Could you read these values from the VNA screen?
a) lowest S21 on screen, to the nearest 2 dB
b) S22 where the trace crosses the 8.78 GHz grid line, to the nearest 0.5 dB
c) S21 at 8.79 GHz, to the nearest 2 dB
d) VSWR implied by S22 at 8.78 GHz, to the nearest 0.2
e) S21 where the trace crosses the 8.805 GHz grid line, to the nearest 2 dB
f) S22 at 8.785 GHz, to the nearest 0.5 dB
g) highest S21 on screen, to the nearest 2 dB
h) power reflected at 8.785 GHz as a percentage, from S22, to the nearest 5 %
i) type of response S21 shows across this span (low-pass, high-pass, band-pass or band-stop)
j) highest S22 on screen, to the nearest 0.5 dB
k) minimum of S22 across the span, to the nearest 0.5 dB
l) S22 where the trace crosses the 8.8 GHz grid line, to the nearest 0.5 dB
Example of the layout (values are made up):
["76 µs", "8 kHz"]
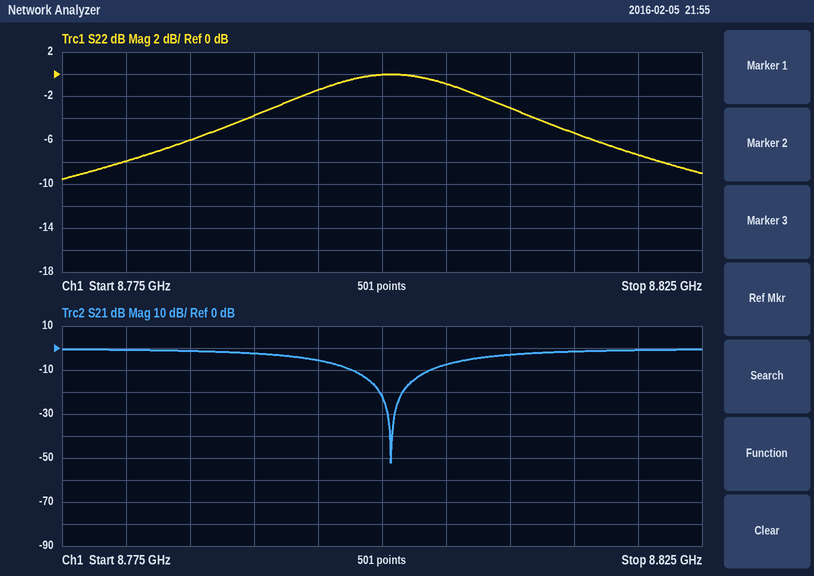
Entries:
["-52 dB", "-8.0 dB", "-2 dB", "2.4", "-8 dB", "-6.0 dB", "0 dB", "25 %", "band-stop", "0.0 dB", "-9.5 dB", "0.0 dB"]
